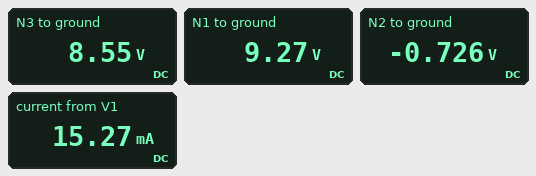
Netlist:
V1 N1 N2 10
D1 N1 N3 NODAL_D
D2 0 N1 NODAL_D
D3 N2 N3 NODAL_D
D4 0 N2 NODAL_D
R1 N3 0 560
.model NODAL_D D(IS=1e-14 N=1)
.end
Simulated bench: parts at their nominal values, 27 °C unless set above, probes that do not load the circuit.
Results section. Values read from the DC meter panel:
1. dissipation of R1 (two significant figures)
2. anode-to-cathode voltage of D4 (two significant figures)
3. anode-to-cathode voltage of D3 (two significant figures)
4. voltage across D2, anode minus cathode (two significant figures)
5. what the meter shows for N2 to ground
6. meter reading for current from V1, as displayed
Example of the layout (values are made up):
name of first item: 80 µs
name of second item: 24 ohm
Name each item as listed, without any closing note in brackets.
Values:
dissipation of R1: 130 mW
anode-to-cathode voltage of D4: 730 mV
anode-to-cathode voltage of D3: -9.3 V
voltage across D2, anode minus cathode: -9.3 V
what the meter shows for N2 to ground: -0.726 V
meter reading for current from V1, as displayed: 15.27 mA
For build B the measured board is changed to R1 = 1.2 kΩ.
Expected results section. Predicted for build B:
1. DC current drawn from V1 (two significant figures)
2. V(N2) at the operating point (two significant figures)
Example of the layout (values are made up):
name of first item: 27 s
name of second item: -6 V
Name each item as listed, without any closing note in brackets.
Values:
DC current drawn from V1: 7.2 mA
V(N2) at the operating point: -710 mV
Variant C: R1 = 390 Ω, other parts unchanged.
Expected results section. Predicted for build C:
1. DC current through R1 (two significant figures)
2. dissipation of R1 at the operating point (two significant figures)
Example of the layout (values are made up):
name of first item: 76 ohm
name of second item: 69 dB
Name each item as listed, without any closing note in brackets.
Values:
DC current through R1: 22 mA
dissipation of R1 at the operating point: 190 mW
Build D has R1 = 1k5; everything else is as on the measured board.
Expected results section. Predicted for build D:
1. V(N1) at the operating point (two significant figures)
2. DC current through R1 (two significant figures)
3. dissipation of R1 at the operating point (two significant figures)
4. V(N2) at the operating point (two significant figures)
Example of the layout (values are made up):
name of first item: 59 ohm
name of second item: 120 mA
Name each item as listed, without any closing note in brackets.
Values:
V(N1) at the operating point: 9.3 V
DC current through R1: 5.7 mA
dissipation of R1 at the operating point: 49 mW
V(N2) at the operating point: -700 mV
